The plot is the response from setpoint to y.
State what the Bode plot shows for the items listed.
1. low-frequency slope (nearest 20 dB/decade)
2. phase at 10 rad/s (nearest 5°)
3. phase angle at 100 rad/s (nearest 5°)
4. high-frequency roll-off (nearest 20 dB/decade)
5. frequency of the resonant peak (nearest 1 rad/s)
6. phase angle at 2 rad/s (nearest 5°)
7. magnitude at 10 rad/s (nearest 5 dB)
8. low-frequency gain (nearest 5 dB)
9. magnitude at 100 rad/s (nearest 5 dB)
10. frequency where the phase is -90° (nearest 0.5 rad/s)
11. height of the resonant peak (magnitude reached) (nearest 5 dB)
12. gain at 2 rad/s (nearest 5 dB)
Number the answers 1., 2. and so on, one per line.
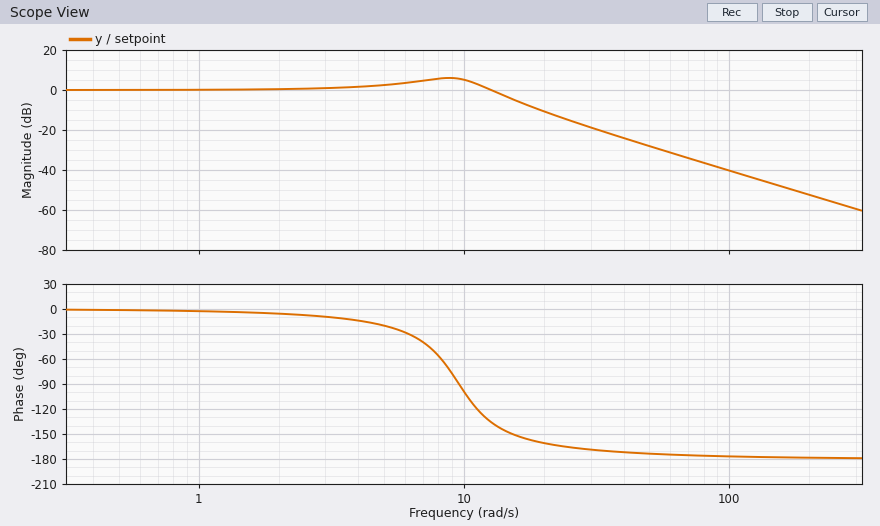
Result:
1. 0 dB/decade
2. -100°
3. -175°
4. -40 dB/decade
5. 9 rad/s
6. -5°
7. 5 dB
8. 0 dB
9. -40 dB
10. 9.5 rad/s
11. 5 dB
12. 0 dB
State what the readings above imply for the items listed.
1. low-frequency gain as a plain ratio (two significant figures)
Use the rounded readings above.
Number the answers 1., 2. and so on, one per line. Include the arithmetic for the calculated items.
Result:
1. 10^(0 / 20) = 1.0
